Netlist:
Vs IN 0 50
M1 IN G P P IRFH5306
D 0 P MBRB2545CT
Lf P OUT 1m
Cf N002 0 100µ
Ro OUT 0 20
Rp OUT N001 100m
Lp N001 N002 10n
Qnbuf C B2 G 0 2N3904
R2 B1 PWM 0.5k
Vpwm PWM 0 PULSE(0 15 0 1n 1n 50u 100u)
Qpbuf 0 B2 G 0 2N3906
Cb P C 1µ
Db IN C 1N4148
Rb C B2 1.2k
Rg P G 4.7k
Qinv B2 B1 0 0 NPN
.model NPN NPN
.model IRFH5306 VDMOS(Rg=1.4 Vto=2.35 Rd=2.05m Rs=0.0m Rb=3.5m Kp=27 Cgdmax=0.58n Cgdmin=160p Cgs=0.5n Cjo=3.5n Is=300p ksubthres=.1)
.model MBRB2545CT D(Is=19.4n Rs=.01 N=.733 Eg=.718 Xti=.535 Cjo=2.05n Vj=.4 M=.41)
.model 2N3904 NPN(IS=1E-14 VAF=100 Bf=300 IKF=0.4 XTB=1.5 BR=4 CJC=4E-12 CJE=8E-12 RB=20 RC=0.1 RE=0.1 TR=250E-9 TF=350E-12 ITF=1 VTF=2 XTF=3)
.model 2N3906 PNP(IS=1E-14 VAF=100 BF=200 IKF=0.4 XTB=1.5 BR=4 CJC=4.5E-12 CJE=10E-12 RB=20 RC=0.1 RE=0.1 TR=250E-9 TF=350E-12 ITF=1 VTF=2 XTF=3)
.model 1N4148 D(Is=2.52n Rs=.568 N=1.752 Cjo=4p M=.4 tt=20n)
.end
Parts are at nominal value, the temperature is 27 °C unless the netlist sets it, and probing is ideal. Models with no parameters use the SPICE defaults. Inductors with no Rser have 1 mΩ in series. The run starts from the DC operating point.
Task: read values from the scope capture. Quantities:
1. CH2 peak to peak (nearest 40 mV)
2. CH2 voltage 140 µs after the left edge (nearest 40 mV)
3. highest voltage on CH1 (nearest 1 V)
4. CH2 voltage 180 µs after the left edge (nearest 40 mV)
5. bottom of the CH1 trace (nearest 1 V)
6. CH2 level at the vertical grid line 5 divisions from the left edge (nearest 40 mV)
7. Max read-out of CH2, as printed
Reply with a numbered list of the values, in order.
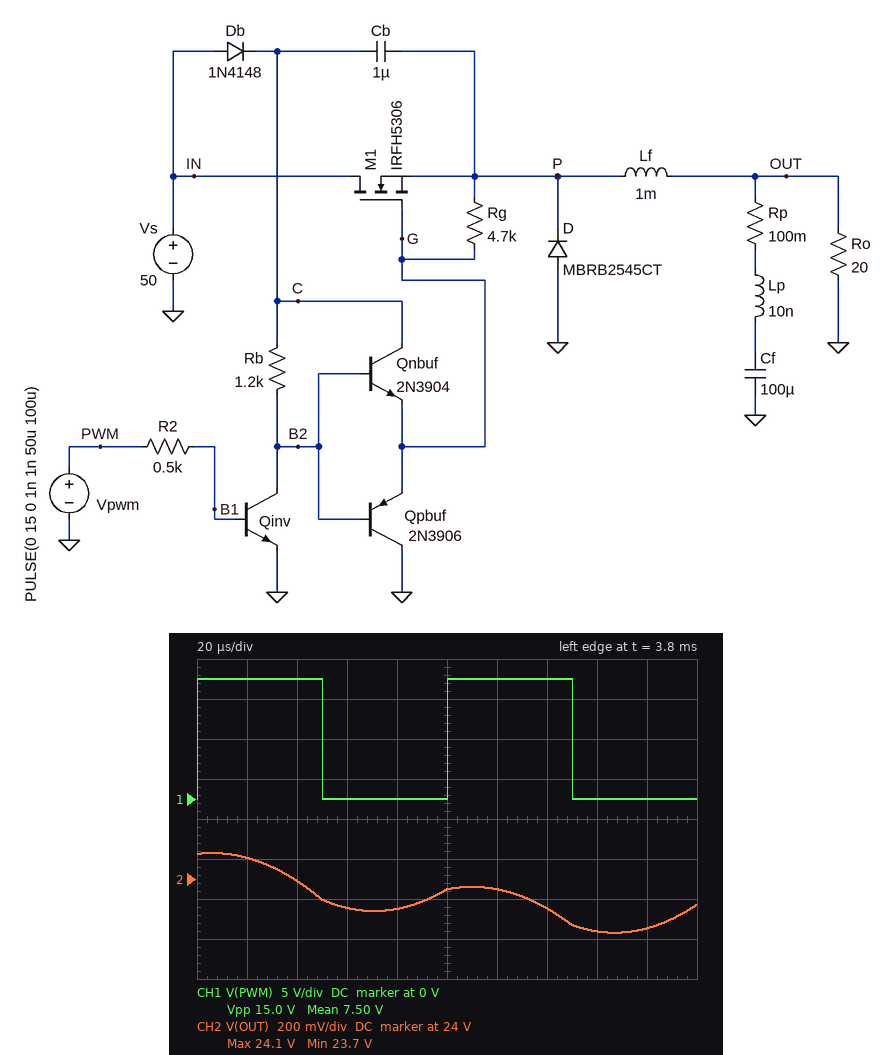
1. 400 mV
2. 23.84 V
3. 15 V
4. 23.76 V
5. 0 V
6. 23.96 V
7. 24.1 V
